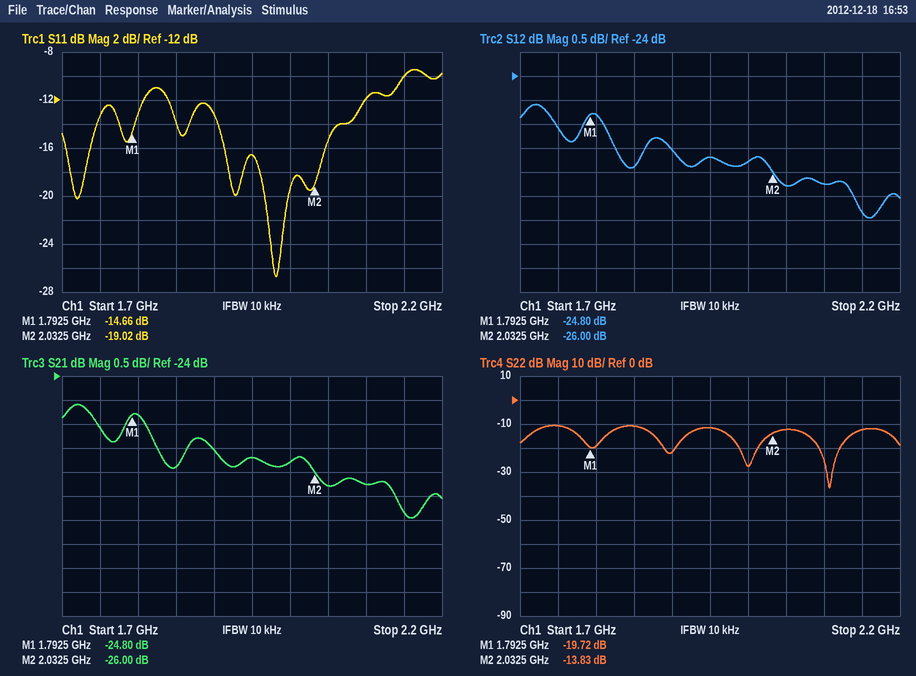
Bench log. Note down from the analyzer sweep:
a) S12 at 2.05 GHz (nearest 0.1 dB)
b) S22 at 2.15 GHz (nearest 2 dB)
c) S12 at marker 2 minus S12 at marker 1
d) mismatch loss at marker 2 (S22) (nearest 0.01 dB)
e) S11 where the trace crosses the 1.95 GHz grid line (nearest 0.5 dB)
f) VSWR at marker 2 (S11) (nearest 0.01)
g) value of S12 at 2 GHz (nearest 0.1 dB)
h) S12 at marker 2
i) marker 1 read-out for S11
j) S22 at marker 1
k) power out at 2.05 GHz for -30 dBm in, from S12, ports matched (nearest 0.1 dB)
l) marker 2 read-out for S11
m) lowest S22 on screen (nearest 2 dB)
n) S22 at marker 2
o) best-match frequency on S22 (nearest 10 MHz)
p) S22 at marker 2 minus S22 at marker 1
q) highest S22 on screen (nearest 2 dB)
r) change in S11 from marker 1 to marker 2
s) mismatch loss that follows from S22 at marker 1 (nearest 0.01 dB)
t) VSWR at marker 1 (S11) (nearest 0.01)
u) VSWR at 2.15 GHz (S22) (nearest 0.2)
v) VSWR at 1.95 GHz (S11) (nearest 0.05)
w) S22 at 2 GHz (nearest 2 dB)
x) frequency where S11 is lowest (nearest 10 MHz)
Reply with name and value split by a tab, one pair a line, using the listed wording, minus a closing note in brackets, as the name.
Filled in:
S12 at 2.05 GHz	-26.3 dB
S22 at 2.15 GHz	-12 dB
S12 at marker 2 minus S12 at marker 1	-1.20 dB
mismatch loss at marker 2 (S22)	0.18 dB
S11 where the trace crosses the 1.95 GHz grid line	-16.5 dB
VSWR at marker 2 (S11)	1.25
value of S12 at 2 GHz	-25.8 dB
S12 at marker 2	-26.00 dB
marker 1 read-out for S11	-14.66 dB
S22 at marker 1	-19.72 dB
power out at 2.05 GHz for -30 dBm in, from S12, ports matched	-56.3 dBm
marker 2 read-out for S11	-19.02 dB
lowest S22 on screen	-36 dB
S22 at marker 2	-13.83 dB
best-match frequency on S22	2.11 GHz
S22 at marker 2 minus S22 at marker 1	5.89 dB
highest S22 on screen	-10 dB
change in S11 from marker 1 to marker 2	-4.36 dB
mismatch loss that follows from S22 at marker 1	0.05 dB
VSWR at marker 1 (S11)	1.45
VSWR at 2.15 GHz (S22)	1.6
VSWR at 1.95 GHz (S11)	1.35
S22 at 2 GHz	-28 dB
frequency where S11 is lowest	1.98 GHz
